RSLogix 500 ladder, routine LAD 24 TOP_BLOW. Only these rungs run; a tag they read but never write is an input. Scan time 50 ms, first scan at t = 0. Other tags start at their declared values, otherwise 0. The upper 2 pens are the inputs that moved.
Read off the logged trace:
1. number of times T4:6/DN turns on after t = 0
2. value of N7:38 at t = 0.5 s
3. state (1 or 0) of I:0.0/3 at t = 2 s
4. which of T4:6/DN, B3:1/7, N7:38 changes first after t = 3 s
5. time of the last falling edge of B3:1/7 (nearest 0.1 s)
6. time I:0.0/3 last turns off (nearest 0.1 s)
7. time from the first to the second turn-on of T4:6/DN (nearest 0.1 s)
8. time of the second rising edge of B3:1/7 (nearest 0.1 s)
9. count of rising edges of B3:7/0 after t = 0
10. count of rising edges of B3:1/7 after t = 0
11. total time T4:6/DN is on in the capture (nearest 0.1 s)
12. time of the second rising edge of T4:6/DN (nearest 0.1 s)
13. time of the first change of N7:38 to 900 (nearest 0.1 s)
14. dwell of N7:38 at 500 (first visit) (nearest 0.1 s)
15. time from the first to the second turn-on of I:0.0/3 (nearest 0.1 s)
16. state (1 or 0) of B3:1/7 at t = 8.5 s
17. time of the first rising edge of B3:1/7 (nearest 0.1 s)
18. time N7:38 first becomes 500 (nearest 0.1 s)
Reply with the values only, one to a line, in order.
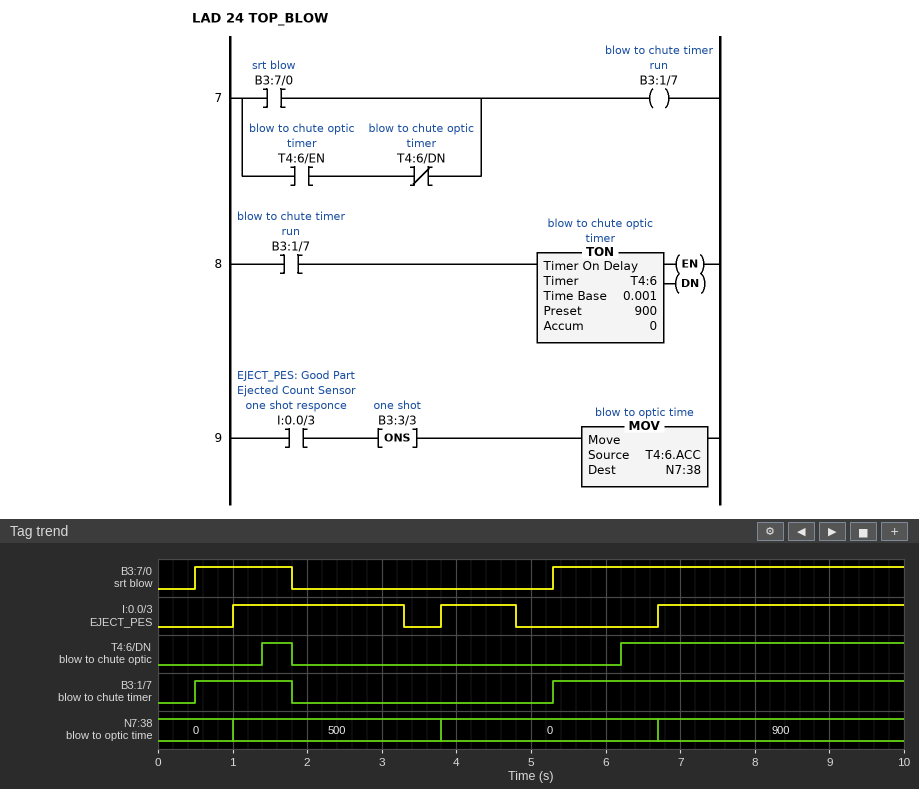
2
0
1
N7:38
1.8 s
4.8 s
4.8 s
5.3 s
2
2
4.2 s
6.2 s
6.7 s
2.8 s
2.8 s
1
0.5 s
1.0 s
